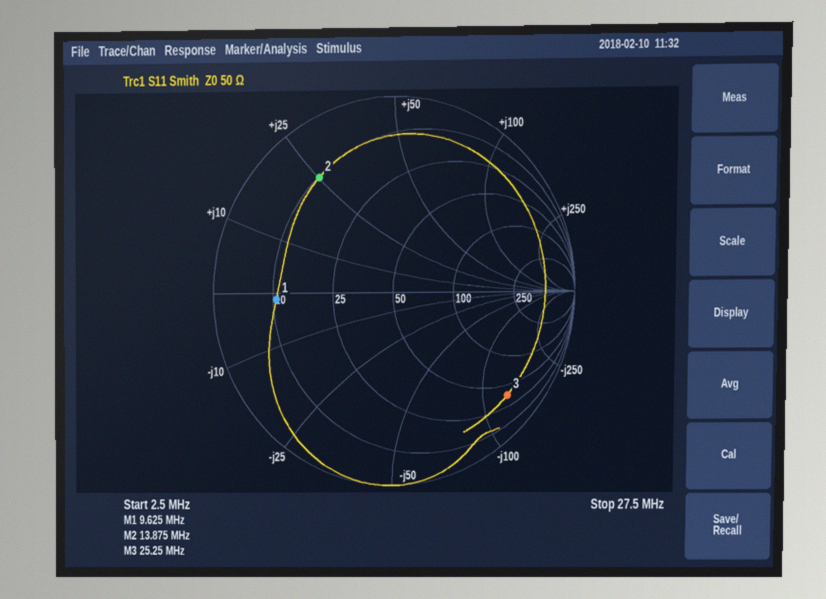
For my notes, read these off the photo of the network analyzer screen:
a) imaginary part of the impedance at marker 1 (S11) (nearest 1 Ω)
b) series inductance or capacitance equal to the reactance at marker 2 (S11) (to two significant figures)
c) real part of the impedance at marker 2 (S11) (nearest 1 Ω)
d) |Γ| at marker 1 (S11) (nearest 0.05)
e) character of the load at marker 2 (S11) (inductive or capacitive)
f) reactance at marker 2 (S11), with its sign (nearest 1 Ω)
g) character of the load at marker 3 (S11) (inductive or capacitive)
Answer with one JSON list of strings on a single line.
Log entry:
["-1 Ω", "290 nH", "10 Ω", "0.65", "inductive", "+25 Ω", "capacitive"]
